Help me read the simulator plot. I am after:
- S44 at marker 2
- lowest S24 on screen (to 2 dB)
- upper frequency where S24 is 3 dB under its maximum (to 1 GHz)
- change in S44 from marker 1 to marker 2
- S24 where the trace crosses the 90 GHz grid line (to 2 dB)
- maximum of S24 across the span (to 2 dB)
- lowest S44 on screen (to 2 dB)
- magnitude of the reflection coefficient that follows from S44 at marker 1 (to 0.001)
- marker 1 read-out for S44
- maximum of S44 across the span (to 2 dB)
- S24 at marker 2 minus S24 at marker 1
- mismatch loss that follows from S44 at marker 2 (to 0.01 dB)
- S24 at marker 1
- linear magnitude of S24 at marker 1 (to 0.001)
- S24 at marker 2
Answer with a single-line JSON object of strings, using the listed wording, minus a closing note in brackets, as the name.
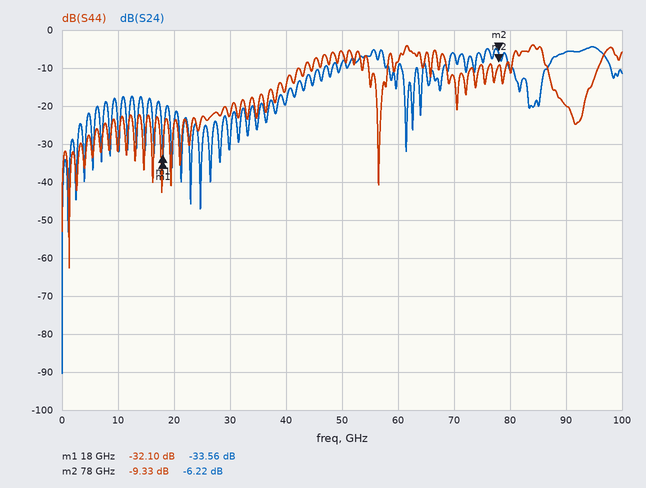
{"S44 at marker 2": "-9.33 dB", "lowest S24 on screen": "-90 dB", "upper frequency where S24 is 3 dB under its maximum": "97 GHz", "change in S44 from marker 1 to marker 2": "22.77 dB", "S24 where the trace crosses the 90 GHz grid line": "-6 dB", "maximum of S24 across the span": "-4 dB", "lowest S44 on screen": "-62 dB", "magnitude of the reflection coefficient that follows from S44 at marker 1": "0.025", "marker 1 read-out for S44": "-32.10 dB", "maximum of S44 across the span": "-4 dB", "S24 at marker 2 minus S24 at marker 1": "27.34 dB", "mismatch loss that follows from S44 at marker 2": "0.54 dB", "S24 at marker 1": "-33.56 dB", "linear magnitude of S24 at marker 1": "0.021", "S24 at marker 2": "-6.22 dB"}
